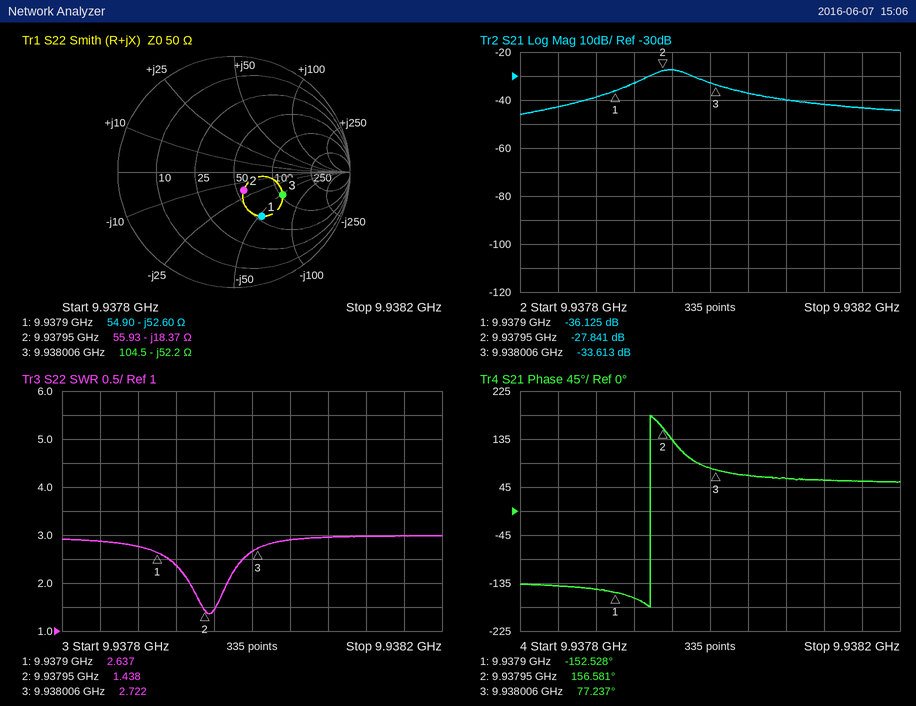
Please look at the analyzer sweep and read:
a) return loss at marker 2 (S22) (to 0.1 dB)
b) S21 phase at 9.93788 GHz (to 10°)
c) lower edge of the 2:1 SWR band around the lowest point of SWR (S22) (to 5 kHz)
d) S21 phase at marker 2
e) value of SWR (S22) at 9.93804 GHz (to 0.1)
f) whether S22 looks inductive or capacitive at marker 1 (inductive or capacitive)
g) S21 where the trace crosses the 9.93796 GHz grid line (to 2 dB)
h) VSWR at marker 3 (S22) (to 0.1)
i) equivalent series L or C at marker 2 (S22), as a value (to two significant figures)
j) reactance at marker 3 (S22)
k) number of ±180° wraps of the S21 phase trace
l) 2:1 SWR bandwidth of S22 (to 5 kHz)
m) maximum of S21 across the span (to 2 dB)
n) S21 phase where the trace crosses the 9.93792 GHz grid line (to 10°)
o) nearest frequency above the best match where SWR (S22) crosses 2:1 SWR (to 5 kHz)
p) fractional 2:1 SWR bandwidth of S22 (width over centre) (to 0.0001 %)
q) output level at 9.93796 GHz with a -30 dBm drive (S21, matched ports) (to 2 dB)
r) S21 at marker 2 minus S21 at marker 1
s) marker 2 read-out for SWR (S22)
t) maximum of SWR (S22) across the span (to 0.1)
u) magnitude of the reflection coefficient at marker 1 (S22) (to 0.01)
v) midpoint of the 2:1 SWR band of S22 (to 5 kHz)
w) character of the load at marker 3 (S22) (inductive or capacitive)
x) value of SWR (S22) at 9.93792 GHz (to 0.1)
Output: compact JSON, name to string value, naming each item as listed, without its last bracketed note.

{"return loss at marker 2 (S22)": "14.9 dB", "S21 phase at 9.93788 GHz": "-150°", "lower edge of the 2:1 SWR band around the lowest point of SWR (S22)": "9.937935 GHz", "S21 phase at marker 2": "156.581°", "value of SWR (S22) at 9.93804 GHz": "2.9", "whether S22 looks inductive or capacitive at marker 1": "capacitive", "S21 where the trace crosses the 9.93796 GHz grid line": "-28 dB", "VSWR at marker 3 (S22)": "2.7", "equivalent series L or C at marker 2 (S22), as a value": "870 fF", "reactance at marker 3": "-52.2 Ω", "number of ±180° wraps of the S21 phase trace": "1", "2:1 SWR bandwidth of S22": "40 kHz", "maximum of S21 across the span": "-28 dB", "S21 phase where the trace crosses the 9.93792 GHz grid line": "-160°", "nearest frequency above the best match where SWR (S22) crosses 2:1 SWR": "9.937975 GHz", "fractional 2:1 SWR bandwidth of S22 (width over centre)": "0.0004 %", "output level at 9.93796 GHz with a -30 dBm drive (S21, matched ports)": "-58 dBm", "S21 at marker 2 minus S21 at marker 1": "8.284 dB", "marker 2 read-out for SWR": "1.438", "maximum of SWR (S22) across the span": "3.0", "magnitude of the reflection coefficient at marker 1 (S22)": "0.45", "midpoint of the 2:1 SWR band of S22": "9.937955 GHz", "character of the load at marker 3 (S22)": "capacitive", "value of SWR (S22) at 9.93792 GHz": "2.4"}
